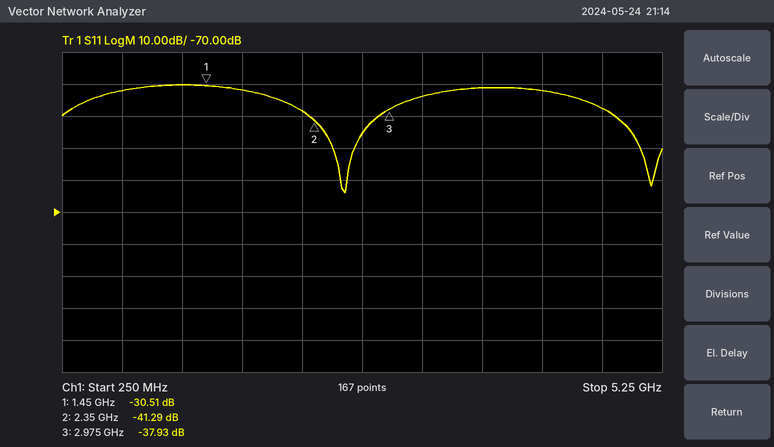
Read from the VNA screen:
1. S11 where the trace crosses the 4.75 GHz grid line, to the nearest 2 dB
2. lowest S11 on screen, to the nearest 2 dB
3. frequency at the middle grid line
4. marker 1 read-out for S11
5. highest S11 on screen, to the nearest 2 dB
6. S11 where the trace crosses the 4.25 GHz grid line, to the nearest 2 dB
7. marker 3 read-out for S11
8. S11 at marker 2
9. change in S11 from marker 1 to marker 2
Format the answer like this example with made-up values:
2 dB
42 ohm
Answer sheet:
-38 dB
-64 dB
2.75 GHz
-30.51 dB
-30 dB
-32 dB
-37.93 dB
-41.29 dB
-10.78 dB
